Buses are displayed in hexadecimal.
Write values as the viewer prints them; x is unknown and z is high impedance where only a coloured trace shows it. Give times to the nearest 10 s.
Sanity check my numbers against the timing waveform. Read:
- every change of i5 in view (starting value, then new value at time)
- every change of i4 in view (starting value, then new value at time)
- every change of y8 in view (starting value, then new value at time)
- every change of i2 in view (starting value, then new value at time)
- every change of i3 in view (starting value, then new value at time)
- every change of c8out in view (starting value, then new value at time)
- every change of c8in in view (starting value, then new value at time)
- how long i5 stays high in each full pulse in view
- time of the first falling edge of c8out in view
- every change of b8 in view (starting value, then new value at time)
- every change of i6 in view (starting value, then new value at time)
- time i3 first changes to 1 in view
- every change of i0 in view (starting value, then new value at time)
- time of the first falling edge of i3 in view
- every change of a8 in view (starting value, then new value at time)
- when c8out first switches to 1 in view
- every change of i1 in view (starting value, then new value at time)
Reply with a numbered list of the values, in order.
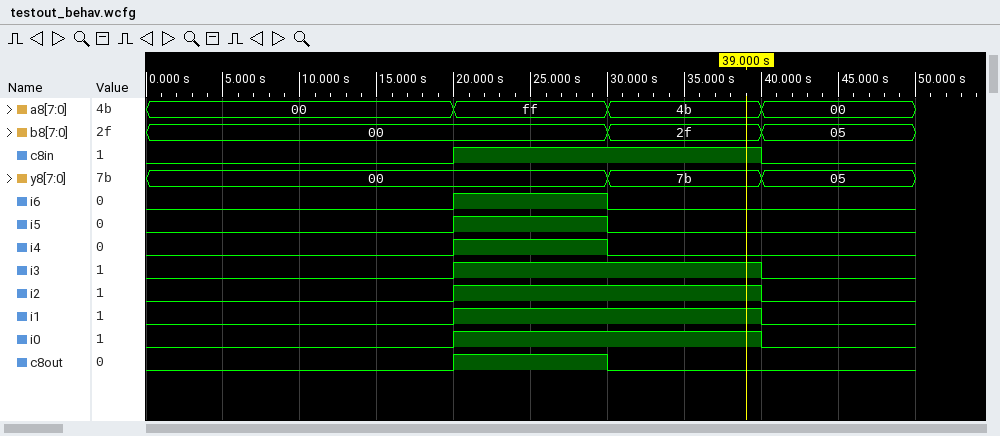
1. 0, 1 at 20 s, 0 at 30 s
2. 0, 1 at 20 s, 0 at 30 s
3. 00, 7b at 30 s, 05 at 40 s
4. 0, 1 at 20 s, 0 at 40 s
5. 0, 1 at 20 s, 0 at 40 s
6. 0, 1 at 20 s, 0 at 30 s
7. 0, 1 at 20 s, 0 at 40 s
8. 10 s
9. 30 s
10. 00, 2f at 30 s, 05 at 40 s
11. 0, 1 at 20 s, 0 at 30 s
12. 20 s
13. 0, 1 at 20 s, 0 at 40 s
14. 40 s
15. 00, ff at 20 s, 4b at 30 s, 00 at 40 s
16. 20 s
17. 0, 1 at 20 s, 0 at 40 s
